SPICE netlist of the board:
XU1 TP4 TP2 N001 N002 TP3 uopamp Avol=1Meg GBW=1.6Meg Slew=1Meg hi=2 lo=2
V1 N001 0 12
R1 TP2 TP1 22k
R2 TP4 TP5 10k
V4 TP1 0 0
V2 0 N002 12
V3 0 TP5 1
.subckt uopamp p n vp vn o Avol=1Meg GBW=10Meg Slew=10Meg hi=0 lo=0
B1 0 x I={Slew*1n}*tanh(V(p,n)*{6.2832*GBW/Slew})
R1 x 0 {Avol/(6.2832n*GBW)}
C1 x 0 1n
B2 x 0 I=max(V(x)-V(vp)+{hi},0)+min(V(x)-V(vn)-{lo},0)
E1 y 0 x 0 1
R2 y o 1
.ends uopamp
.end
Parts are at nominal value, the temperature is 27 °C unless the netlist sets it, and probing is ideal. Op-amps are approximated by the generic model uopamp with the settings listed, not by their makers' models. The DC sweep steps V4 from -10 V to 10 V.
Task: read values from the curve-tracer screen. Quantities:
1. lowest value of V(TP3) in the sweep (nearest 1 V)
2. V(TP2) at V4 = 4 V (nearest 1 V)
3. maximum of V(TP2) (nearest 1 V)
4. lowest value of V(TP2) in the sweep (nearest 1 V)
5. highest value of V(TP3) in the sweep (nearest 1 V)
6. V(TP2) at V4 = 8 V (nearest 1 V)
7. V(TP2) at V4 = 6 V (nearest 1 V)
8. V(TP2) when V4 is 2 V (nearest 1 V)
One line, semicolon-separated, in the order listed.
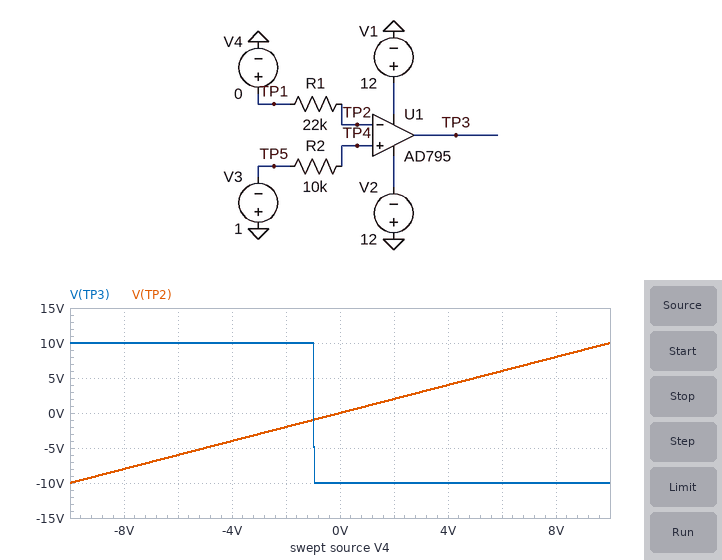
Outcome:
-10 V; 4 V; 10 V; -10 V; 10 V; 8 V; 6 V; 2 V
